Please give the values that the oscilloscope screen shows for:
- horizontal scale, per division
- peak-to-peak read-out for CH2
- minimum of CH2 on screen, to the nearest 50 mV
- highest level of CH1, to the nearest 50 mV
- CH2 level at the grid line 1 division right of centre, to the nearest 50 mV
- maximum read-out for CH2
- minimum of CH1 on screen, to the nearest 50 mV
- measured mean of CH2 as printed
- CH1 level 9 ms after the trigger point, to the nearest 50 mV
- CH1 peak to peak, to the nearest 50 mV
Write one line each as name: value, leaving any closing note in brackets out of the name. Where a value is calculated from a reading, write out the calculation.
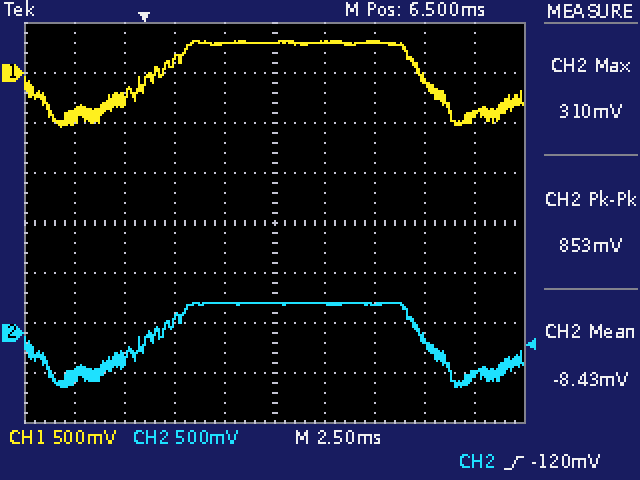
horizontal scale, per division: 2.5 ms
peak-to-peak read-out for CH2: 853 mV
minimum of CH2 on screen, to the nearest 50 mV: -550 mV
highest level of CH1, to the nearest 50 mV: 300 mV
CH2 level at the grid line 1 division right of centre, to the nearest 50 mV: 300 mV
maximum read-out for CH2: 310 mV
minimum of CH1 on screen, to the nearest 50 mV: -550 mV
measured mean of CH2 as printed: -8.43 mV
CH1 level 9 ms after the trigger point, to the nearest 50 mV: 300 mV
CH1 peak to peak, to the nearest 50 mV: 300 mV − (-550 mV) = 850 mV
